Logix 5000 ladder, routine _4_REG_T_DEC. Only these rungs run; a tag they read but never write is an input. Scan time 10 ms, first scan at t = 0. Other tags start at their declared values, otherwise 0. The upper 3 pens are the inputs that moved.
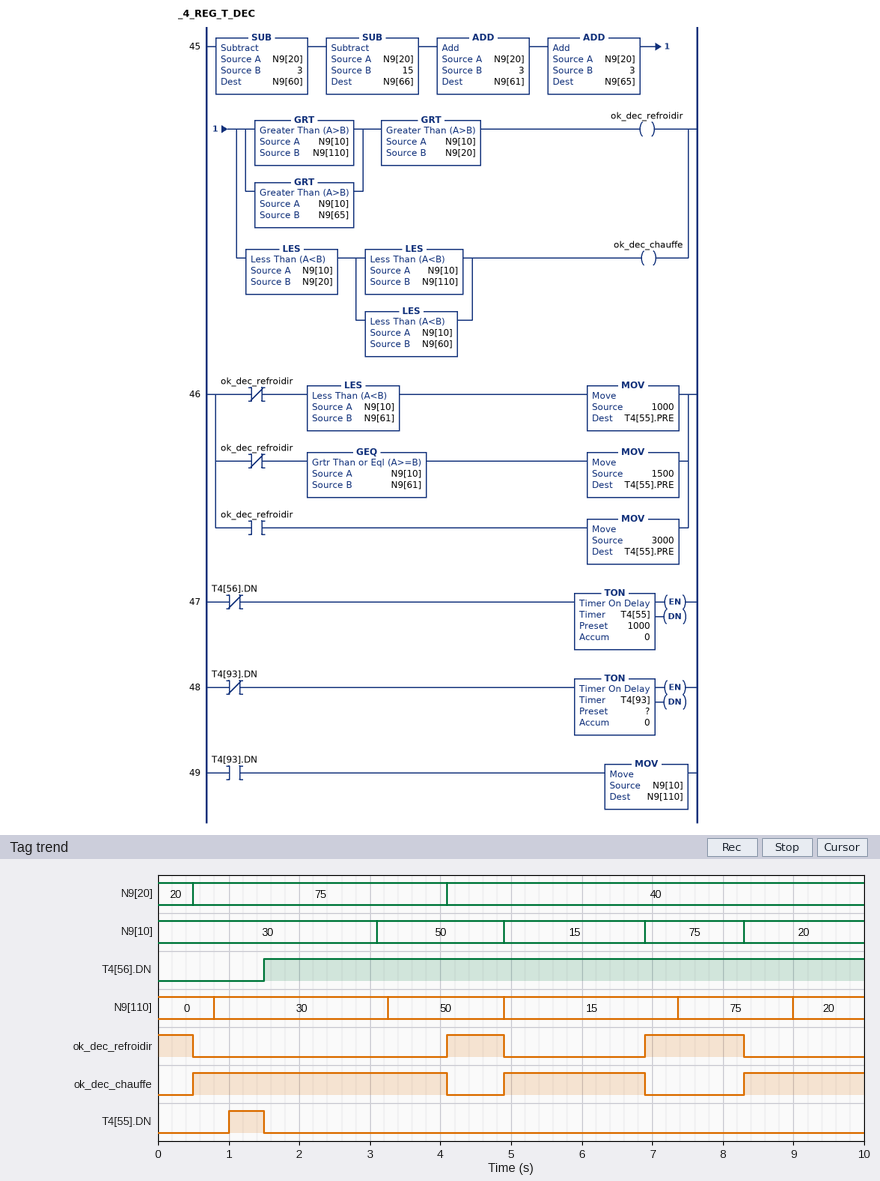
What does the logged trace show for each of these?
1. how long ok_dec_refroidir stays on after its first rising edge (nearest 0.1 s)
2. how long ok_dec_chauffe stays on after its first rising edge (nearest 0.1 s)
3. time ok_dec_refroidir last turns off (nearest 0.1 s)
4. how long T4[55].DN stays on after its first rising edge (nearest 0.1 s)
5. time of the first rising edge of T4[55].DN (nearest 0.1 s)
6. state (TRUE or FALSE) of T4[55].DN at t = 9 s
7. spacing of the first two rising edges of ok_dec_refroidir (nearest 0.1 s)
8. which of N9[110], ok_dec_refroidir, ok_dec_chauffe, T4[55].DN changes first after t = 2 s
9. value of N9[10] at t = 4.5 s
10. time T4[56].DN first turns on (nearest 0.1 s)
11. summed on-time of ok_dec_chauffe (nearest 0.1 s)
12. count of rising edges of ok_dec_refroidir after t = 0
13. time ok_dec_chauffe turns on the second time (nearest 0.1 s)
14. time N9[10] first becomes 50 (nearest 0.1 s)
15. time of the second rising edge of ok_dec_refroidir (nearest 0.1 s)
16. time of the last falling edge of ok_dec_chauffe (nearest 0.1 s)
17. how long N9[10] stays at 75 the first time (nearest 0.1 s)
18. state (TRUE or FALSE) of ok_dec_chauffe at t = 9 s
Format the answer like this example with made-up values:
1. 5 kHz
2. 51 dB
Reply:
1. 0.8 s
2. 3.6 s
3. 8.3 s
4. 0.5 s
5. 1.0 s
6. FALSE
7. 2.8 s
8. N9[110]
9. 50
10. 1.5 s
11. 7.3 s
12. 2
13. 4.9 s
14. 3.1 s
15. 6.9 s
16. 6.9 s
17. 1.4 s
18. TRUE
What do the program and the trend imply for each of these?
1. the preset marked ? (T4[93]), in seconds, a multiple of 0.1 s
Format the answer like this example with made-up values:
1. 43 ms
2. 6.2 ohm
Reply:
1. 0.8 s
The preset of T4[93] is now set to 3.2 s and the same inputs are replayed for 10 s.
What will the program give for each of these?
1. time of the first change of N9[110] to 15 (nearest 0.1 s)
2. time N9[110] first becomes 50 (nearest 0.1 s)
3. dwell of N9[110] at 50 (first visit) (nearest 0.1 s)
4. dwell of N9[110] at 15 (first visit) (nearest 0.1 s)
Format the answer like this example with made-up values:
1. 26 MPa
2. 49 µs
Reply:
1. 6.4 s
2. 3.2 s
3. 3.2 s
4. 3.2 s
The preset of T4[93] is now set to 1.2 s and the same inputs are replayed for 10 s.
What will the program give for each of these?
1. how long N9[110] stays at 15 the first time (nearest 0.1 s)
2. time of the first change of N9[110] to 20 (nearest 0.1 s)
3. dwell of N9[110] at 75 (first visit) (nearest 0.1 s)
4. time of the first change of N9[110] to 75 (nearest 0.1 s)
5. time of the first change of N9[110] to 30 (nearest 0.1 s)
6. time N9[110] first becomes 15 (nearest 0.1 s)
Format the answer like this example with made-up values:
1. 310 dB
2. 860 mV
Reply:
1. 1.2 s
2. 8.5 s
3. 1.2 s
4. 7.3 s
5. 1.2 s
6. 6.1 s
